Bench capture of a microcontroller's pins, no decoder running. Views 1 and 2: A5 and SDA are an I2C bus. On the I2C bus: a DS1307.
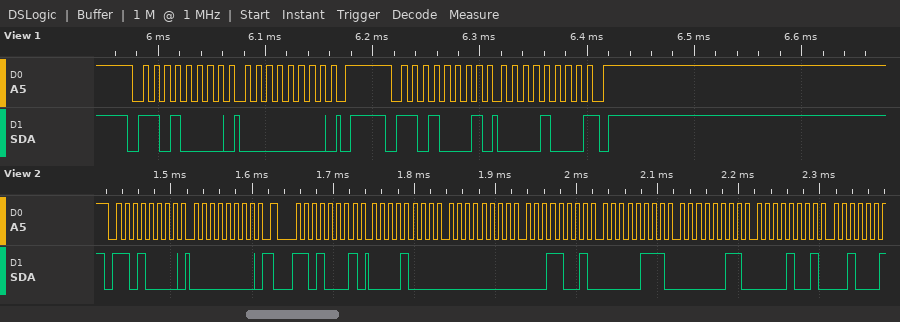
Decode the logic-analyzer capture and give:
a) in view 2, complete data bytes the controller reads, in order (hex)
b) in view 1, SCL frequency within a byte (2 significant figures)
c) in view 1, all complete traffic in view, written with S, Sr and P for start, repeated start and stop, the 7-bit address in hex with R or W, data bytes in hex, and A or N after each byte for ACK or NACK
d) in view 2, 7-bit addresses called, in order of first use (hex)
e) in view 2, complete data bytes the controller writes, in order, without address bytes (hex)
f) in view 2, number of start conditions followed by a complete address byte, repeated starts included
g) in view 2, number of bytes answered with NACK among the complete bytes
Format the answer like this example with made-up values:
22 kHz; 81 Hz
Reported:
08 00 19 07 03 09; 100 kHz; S 68W A 00 A P S 68R A 08 N P; 0x68; 00; 2; 0
